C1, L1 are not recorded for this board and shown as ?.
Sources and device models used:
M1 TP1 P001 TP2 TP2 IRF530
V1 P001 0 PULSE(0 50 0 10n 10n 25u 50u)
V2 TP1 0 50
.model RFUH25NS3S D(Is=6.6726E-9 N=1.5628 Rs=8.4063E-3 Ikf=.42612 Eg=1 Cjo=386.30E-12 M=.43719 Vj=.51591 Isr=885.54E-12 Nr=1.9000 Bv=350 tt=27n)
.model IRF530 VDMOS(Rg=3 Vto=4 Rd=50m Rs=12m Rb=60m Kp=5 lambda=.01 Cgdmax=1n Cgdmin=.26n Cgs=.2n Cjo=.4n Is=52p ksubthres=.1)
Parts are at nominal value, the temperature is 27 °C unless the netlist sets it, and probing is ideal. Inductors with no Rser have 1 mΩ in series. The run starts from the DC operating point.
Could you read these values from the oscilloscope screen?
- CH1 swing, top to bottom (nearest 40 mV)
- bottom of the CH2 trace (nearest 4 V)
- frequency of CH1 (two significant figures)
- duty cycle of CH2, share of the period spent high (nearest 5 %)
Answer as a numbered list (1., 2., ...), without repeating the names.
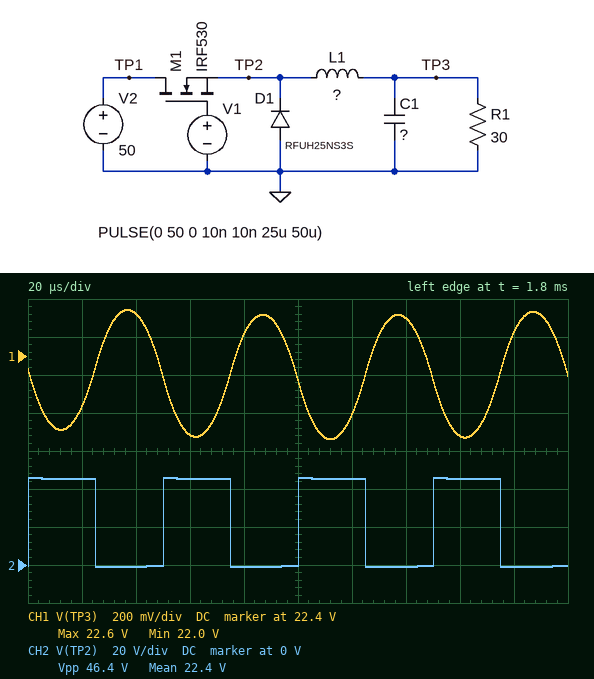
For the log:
1. 680 mV
2. 0 V
3. 20 kHz
4. 50 %
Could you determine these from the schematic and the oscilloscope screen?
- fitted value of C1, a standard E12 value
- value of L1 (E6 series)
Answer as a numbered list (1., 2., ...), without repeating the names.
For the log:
1. 5.6 µF
2. 1 mH
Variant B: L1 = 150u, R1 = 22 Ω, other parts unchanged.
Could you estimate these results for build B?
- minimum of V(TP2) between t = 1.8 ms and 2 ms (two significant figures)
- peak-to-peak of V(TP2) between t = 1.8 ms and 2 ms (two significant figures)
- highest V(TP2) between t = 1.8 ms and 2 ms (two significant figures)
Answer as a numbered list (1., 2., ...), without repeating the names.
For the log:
1. -920 mV
2. 52 V
3. 51 V
